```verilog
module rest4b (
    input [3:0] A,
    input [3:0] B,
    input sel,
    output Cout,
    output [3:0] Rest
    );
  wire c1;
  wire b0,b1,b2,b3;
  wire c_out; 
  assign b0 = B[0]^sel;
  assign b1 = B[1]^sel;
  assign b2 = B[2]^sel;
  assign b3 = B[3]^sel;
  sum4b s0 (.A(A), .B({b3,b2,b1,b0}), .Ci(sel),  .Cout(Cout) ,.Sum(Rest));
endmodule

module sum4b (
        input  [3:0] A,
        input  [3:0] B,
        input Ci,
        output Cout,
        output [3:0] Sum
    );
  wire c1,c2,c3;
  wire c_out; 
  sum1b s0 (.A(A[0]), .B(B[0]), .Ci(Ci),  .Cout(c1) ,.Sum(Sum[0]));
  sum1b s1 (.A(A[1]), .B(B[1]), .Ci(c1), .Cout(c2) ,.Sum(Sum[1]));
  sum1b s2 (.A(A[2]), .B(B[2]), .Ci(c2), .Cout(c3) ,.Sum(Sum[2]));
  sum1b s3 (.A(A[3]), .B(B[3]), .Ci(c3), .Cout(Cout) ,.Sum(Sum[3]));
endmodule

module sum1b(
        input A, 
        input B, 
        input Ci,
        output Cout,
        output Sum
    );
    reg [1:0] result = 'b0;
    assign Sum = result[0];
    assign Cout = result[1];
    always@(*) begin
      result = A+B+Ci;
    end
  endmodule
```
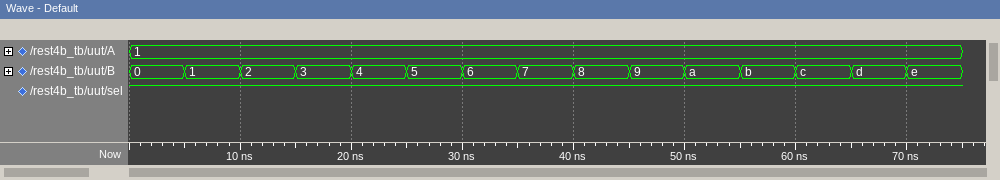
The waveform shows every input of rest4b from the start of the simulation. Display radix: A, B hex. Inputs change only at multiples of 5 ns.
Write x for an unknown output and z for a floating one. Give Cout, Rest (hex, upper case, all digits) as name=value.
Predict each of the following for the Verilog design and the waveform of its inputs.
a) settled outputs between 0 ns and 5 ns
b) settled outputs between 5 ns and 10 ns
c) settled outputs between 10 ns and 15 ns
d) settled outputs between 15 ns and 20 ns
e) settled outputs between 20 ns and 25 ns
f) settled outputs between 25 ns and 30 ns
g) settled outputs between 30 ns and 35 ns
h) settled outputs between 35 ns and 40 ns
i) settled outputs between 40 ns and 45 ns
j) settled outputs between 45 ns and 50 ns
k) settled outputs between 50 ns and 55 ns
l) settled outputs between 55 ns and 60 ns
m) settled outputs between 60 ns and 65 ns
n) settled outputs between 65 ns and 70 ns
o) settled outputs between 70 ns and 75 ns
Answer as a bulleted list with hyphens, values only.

- Cout=1, Rest=1
- Cout=1, Rest=0
- Cout=0, Rest=F
- Cout=0, Rest=E
- Cout=0, Rest=D
- Cout=0, Rest=C
- Cout=0, Rest=B
- Cout=0, Rest=A
- Cout=0, Rest=9
- Cout=0, Rest=8
- Cout=0, Rest=7
- Cout=0, Rest=6
- Cout=0, Rest=5
- Cout=0, Rest=4
- Cout=0, Rest=3
